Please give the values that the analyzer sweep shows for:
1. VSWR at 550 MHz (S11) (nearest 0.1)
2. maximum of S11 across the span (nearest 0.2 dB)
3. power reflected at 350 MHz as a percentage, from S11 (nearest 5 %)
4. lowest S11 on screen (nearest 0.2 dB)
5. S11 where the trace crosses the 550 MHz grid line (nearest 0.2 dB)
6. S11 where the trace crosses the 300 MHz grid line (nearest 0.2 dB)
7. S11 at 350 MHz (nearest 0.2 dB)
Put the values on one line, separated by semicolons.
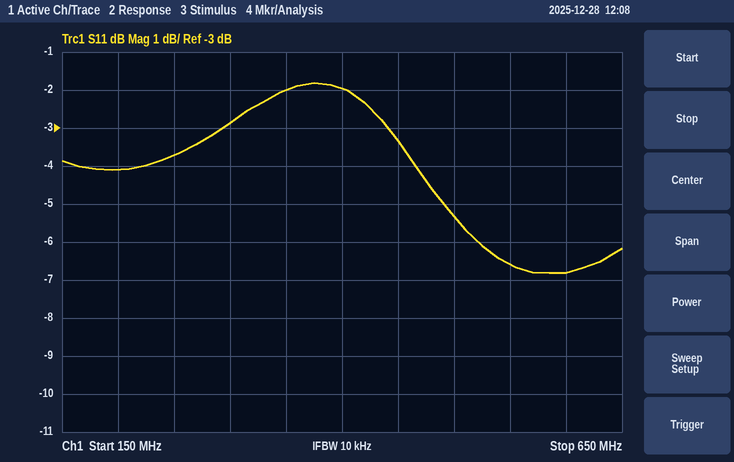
2.8; -1.8 dB; 65 %; -6.8 dB; -6.6 dB; -2.8 dB; -2.0 dB
